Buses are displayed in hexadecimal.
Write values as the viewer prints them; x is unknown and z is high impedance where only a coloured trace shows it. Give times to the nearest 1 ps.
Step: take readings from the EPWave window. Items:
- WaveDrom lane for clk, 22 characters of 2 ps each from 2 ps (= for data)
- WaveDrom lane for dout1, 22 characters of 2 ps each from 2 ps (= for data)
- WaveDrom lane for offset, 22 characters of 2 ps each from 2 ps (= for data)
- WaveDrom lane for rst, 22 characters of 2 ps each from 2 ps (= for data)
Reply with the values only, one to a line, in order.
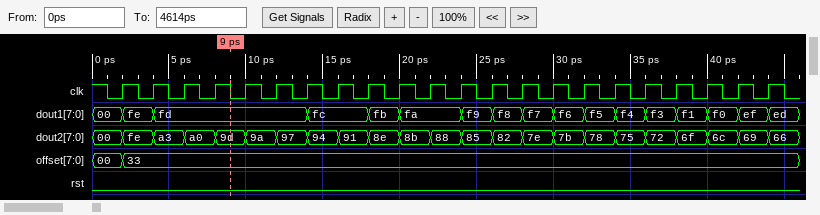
{name: 'clk', wave: 'p.....................'}
{name: 'dout1', wave: '==....=.==.===========', data: 'fe fd fc fb fa f9 f8 f7 f6 f5 f4 f3 f1 f0 ef ed'}
{name: 'offset', wave: '=.....................', data: '33'}
{name: 'rst', wave: '0.....................'}
